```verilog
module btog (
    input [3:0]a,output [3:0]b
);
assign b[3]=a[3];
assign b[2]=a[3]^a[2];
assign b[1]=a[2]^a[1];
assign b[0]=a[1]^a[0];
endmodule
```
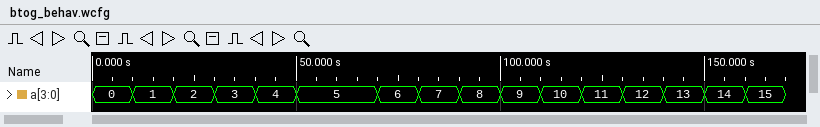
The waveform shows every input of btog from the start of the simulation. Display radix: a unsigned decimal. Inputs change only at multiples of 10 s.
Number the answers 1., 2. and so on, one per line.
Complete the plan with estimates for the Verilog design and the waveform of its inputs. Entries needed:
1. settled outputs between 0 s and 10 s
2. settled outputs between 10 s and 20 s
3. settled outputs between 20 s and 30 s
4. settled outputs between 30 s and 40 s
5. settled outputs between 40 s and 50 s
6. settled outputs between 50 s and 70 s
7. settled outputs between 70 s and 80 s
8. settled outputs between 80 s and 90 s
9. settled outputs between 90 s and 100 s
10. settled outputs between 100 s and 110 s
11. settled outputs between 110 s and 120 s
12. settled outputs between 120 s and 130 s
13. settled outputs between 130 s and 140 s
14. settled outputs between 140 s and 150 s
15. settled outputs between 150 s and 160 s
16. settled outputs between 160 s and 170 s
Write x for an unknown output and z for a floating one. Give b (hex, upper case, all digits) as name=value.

1. b=0
2. b=1
3. b=3
4. b=2
5. b=6
6. b=7
7. b=5
8. b=4
9. b=C
10. b=D
11. b=F
12. b=E
13. b=A
14. b=B
15. b=9
16. b=8
